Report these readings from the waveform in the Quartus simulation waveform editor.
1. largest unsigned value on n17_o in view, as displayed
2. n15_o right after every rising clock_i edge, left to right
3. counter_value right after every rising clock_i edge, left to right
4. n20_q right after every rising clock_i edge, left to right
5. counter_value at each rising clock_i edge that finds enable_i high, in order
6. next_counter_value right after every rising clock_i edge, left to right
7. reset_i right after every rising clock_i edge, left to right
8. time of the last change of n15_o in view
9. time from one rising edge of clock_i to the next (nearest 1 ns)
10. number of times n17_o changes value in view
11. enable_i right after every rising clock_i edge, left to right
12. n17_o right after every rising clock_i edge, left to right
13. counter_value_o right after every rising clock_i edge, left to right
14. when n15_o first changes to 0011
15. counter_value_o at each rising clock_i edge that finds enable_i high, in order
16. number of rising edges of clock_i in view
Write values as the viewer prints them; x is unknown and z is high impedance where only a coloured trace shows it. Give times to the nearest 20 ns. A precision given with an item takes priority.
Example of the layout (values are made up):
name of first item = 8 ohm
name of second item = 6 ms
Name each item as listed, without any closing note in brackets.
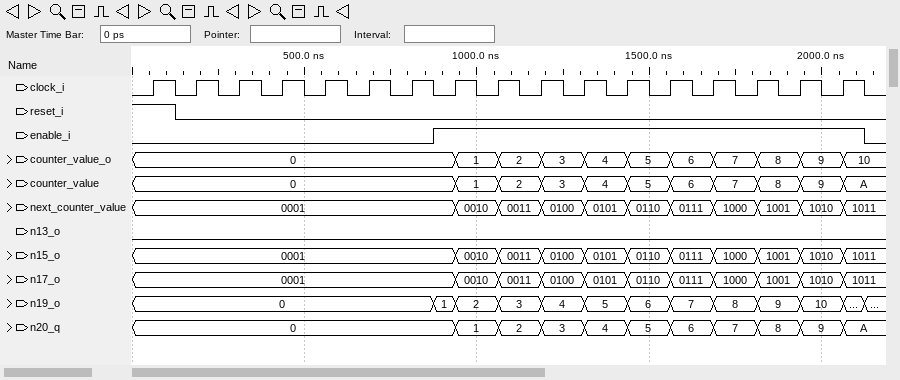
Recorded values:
largest unsigned value on n17_o in view, as displayed = 1011
n15_o right after every rising clock_i edge, left to right = 0001, 0001, 0001, 0001, 0001, 0001, 0001, 0010, 0011, 0100, 0101, 0110, 0111, 1000, 1001, 1010, 1011
counter_value right after every rising clock_i edge, left to right = 0, 0, 0, 0, 0, 0, 0, 1, 2, 3, 4, 5, 6, 7, 8, 9, A
n20_q right after every rising clock_i edge, left to right = 0, 0, 0, 0, 0, 0, 0, 1, 2, 3, 4, 5, 6, 7, 8, 9, A
counter_value at each rising clock_i edge that finds enable_i high, in order = 0, 1, 2, 3, 4, 5, 6, 7, 8, 9
next_counter_value right after every rising clock_i edge, left to right = 0001, 0001, 0001, 0001, 0001, 0001, 0001, 0010, 0011, 0100, 0101, 0110, 0111, 1000, 1001, 1010, 1011
reset_i right after every rising clock_i edge, left to right = 1 0 0 0 0 0 0 0 0 0 0 0 0 0 0 0 0
time of the last change of n15_o in view = 2060 ns
time from one rising edge of clock_i to the next = 125 ns
number of times n17_o changes value in view = 10
enable_i right after every rising clock_i edge, left to right = 0 0 0 0 0 0 0 1 1 1 1 1 1 1 1 1 1
n17_o right after every rising clock_i edge, left to right = 0001, 0001, 0001, 0001, 0001, 0001, 0001, 0010, 0011, 0100, 0101, 0110, 0111, 1000, 1001, 1010, 1011
counter_value_o right after every rising clock_i edge, left to right = 0, 0, 0, 0, 0, 0, 0, 1, 2, 3, 4, 5, 6, 7, 8, 9, 10
when n15_o first changes to 0011 = 1060 ns
counter_value_o at each rising clock_i edge that finds enable_i high, in order = 0, 1, 2, 3, 4, 5, 6, 7, 8, 9
number of rising edges of clock_i in view = 17
